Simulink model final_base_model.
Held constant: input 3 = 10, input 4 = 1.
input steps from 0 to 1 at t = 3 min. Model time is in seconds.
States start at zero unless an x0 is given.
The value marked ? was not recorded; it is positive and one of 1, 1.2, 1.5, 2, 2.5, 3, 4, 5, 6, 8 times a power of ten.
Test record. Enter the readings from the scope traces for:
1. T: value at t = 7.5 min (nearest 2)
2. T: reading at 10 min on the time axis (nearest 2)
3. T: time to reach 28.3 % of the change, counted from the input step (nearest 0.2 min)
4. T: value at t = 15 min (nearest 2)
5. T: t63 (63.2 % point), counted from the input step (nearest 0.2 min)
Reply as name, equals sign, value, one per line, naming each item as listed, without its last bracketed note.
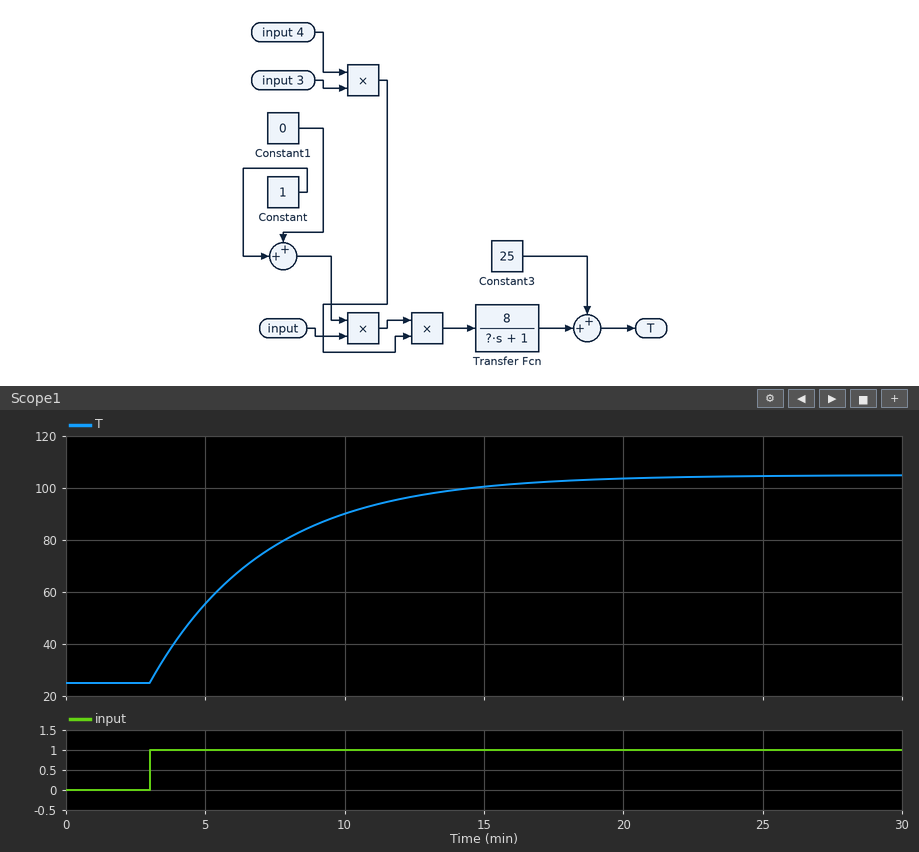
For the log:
T: value at t = 7.5 min = 78
T: reading at 10 min on the time axis = 90
T: time to reach 28.3 % of the change, counted from the input step = 1.4 min
T: value at t = 15 min = 100
T: t63 (63.2 % point), counted from the input step = 4.2 min
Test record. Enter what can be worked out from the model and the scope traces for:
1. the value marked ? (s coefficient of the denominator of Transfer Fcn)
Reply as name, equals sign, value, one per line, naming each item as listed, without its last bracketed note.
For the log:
the value marked ? = 250
